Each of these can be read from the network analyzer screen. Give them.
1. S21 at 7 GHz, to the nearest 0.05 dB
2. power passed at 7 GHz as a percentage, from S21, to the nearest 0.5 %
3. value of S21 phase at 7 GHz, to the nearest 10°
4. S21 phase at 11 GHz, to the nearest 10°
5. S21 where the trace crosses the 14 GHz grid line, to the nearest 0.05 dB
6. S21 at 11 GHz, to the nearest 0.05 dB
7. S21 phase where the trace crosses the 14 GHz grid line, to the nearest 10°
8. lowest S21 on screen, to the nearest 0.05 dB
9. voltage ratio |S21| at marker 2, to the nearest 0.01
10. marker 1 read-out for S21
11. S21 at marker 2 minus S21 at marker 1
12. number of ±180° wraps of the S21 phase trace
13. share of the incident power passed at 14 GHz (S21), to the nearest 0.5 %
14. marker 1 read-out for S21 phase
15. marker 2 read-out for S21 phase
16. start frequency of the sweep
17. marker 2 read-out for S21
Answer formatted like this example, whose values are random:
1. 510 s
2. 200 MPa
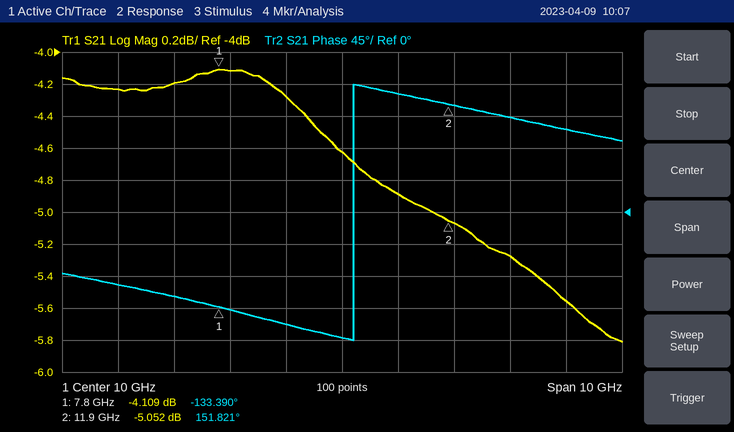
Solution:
1. -4.20 dB
2. 38.0 %
3. -120°
4. 170°
5. -5.55 dB
6. -4.90 dB
7. 120°
8. -5.80 dB
9. 0.56
10. -4.109 dB
11. -0.943 dB
12. 1
13. 28.0 %
14. -133.390°
15. 151.821°
16. 5 GHz
17. -5.052 dB
